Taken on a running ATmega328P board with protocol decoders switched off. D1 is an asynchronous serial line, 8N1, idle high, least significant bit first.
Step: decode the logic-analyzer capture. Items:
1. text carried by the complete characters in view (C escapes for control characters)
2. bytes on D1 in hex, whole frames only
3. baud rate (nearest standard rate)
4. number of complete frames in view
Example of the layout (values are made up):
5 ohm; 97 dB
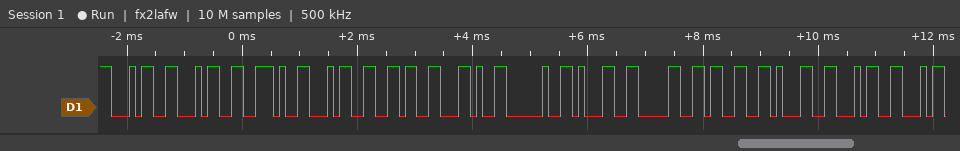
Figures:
"44.46, 10314"; 34 34 2E 34 36 2C 20 31 30 33 31 34; 9600 baud; 12
